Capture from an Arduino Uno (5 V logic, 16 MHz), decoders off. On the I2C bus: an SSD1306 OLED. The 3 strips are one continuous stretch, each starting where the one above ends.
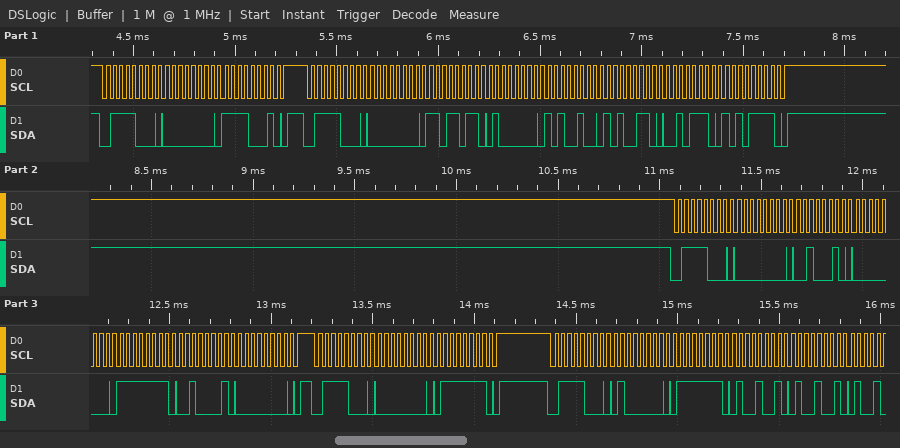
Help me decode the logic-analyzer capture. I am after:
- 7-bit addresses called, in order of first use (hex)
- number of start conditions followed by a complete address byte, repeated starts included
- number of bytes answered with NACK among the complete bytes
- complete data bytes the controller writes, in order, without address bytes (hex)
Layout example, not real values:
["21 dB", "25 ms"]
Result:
["0x3C", "5", "0", "00 F1 00 DB 40 A4 A6 2E AF 00 22 00 FF 21 00 00 7F 40 7F 49 49"]
